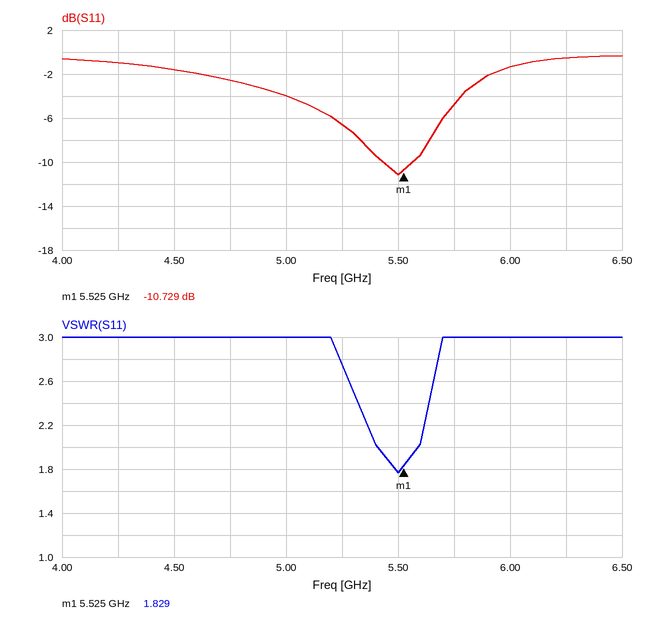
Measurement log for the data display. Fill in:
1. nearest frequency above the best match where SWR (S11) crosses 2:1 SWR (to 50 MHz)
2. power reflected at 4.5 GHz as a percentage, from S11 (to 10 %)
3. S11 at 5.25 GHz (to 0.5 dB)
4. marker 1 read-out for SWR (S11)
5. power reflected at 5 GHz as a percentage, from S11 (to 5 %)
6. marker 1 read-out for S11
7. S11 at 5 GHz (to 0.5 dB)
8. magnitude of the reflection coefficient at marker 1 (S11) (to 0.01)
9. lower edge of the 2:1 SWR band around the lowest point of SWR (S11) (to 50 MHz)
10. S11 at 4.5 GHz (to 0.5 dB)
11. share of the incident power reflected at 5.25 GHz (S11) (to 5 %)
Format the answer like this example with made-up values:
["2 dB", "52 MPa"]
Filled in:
["5.60 GHz", "70 %", "-6.5 dB", "1.829", "40 %", "-10.729 dB", "-4.0 dB", "0.29", "5.40 GHz", "-1.5 dB", "20 %"]
